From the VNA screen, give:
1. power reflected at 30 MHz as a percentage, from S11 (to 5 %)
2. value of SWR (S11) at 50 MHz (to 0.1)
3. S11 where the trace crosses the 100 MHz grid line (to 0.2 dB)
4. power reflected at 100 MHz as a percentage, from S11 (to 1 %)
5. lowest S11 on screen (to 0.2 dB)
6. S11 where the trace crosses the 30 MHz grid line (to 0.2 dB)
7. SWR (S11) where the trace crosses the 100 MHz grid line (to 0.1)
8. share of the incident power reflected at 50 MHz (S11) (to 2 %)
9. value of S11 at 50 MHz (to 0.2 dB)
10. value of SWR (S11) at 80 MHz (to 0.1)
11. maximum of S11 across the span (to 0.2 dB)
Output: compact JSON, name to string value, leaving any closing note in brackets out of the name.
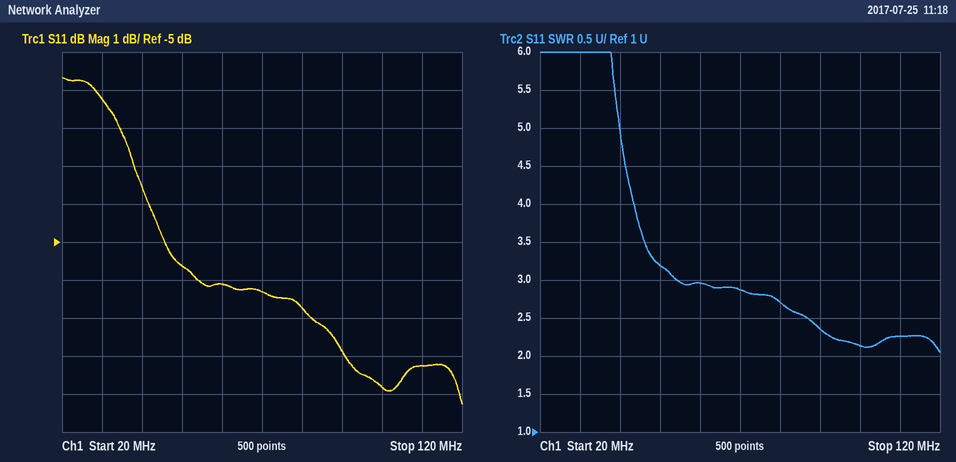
{"power reflected at 30 MHz as a percentage, from S11": "75 %", "value of SWR (S11) at 50 MHz": "3.2", "S11 where the trace crosses the 100 MHz grid line": "-8.8 dB", "power reflected at 100 MHz as a percentage, from S11": "13 %", "lowest S11 on screen": "-9.2 dB", "S11 where the trace crosses the 30 MHz grid line": "-1.2 dB", "SWR (S11) where the trace crosses the 100 MHz grid line": "2.1", "share of the incident power reflected at 50 MHz (S11)": "28 %", "value of S11 at 50 MHz": "-5.6 dB", "value of SWR (S11) at 80 MHz": "2.7", "maximum of S11 across the span": "-0.6 dB"}
